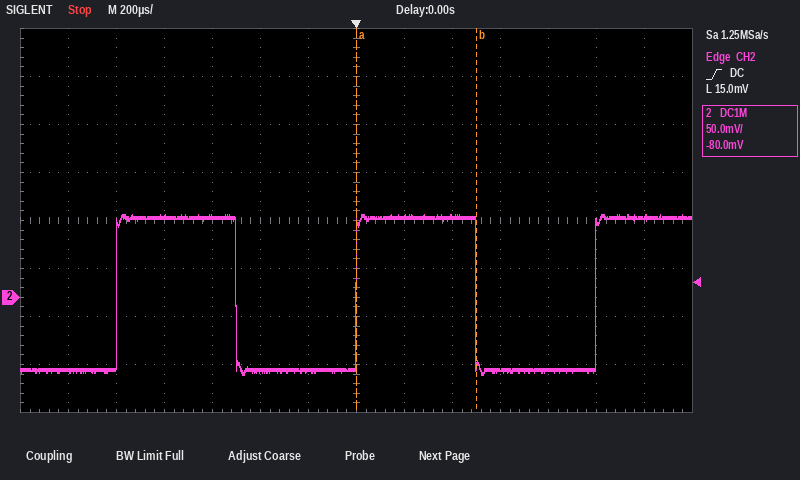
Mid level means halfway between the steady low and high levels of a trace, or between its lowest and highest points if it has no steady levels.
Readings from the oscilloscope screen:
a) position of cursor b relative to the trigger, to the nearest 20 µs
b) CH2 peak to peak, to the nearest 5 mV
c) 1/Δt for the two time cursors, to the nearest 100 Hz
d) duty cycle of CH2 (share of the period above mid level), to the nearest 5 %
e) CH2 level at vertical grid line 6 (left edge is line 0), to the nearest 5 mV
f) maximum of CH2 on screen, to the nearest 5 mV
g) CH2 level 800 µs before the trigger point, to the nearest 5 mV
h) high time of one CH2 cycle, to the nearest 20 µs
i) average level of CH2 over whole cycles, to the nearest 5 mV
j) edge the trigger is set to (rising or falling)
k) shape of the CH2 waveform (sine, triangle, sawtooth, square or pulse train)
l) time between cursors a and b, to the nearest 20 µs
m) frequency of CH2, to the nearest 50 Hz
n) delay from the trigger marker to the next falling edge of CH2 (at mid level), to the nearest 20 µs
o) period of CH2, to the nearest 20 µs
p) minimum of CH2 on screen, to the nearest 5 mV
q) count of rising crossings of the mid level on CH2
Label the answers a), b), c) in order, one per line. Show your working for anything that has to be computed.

a) +500 µs
b) 85 mV − (-80 mV) = 165 mV
c) 1 / 500 µs ≈ 2.0 kHz
d) 500 µs / 1.00 ms ≈ 50 %
e) -75 mV
f) 85 mV
g) 85 mV
h) 500 µs
i) -80 mV + 0.5 × (85 mV − (-80 mV)) ≈ 2.50 mV, so 5 mV to the nearest 5 mV
j) rising
k) square
l) 500 µs
m) 1 / 1.00 ms ≈ 1.00 kHz
n) 500 µs
o) 1.00 ms
p) -80 mV
q) 3
